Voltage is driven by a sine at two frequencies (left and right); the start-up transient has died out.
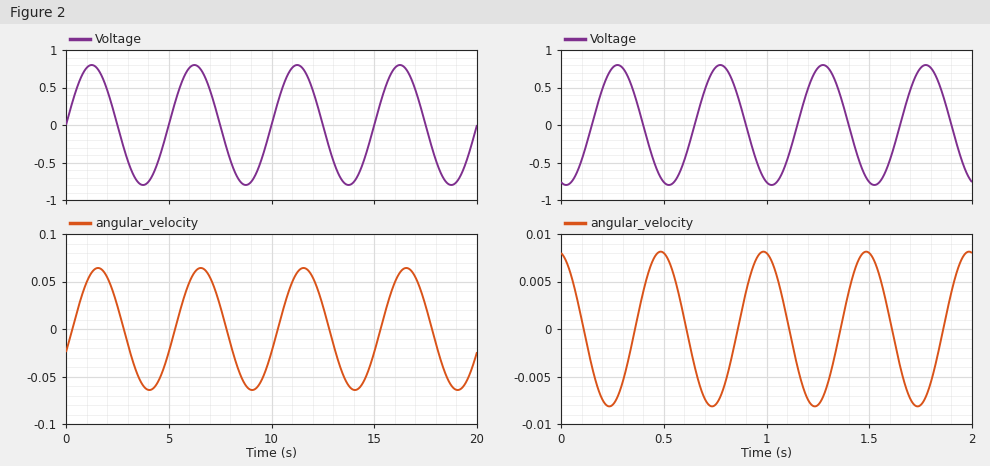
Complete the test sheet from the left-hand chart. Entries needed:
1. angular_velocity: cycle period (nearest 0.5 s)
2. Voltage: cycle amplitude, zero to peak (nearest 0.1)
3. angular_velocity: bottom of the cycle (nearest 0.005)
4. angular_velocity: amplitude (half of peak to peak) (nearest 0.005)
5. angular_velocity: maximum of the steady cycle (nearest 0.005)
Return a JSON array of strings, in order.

["5.0 s", "0.8", "-0.065", "0.065", "0.065"]
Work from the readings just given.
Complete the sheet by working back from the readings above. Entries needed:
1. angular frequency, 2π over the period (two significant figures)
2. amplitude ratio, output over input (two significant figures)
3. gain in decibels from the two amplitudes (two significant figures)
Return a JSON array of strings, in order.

["1.3 rad/s", "0.081", "-22 dB"]
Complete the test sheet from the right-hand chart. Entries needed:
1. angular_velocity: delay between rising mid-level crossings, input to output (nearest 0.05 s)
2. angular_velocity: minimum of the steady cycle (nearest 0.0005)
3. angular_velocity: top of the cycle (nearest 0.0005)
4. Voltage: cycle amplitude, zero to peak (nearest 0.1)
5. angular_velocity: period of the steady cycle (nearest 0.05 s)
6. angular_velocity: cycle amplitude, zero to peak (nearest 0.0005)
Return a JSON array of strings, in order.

["0.20 s", "-0.0080", "0.0080", "0.8", "0.50 s", "0.0080"]
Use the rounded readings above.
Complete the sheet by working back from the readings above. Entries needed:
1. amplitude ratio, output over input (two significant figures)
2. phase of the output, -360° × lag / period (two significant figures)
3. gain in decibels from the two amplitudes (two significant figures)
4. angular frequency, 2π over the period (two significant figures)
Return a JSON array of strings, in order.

["0.010", "-140°", "-40 dB", "13 rad/s"]
